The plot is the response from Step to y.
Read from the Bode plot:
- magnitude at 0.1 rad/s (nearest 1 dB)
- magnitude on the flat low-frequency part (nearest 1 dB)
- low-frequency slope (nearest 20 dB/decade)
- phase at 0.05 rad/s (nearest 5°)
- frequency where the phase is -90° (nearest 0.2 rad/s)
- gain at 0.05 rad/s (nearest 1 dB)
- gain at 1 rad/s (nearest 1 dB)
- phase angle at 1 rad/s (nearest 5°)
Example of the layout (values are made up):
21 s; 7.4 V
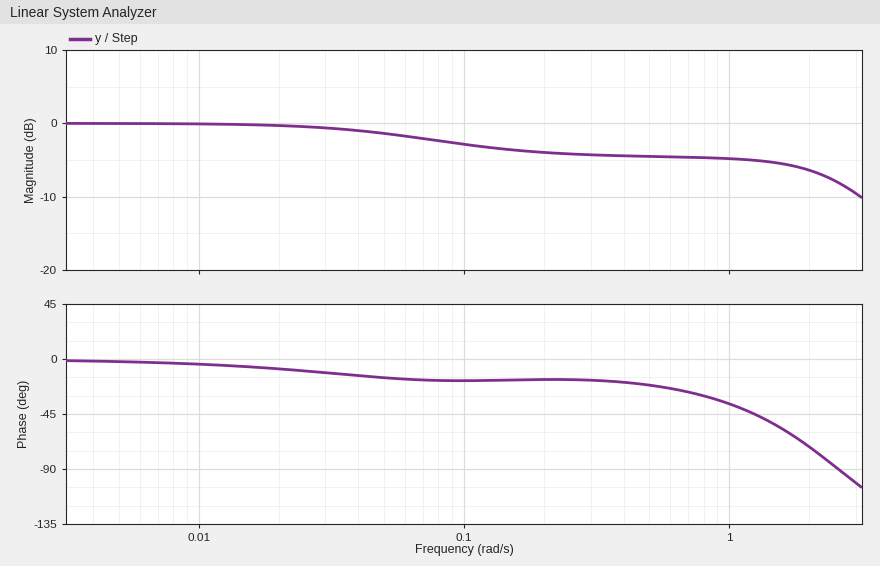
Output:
-3 dB; 0 dB; 0 dB/decade; -15°; 2.6 rad/s; -1 dB; -5 dB; -35°
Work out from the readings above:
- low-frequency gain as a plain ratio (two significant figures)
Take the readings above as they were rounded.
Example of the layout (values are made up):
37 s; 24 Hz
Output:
1.0
